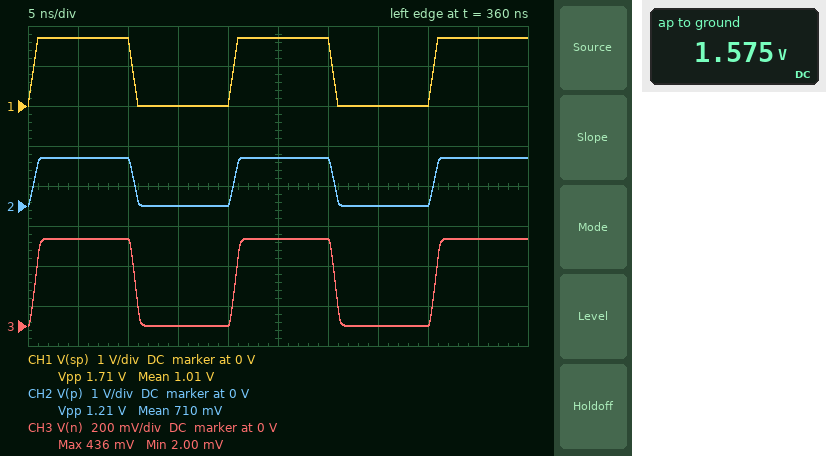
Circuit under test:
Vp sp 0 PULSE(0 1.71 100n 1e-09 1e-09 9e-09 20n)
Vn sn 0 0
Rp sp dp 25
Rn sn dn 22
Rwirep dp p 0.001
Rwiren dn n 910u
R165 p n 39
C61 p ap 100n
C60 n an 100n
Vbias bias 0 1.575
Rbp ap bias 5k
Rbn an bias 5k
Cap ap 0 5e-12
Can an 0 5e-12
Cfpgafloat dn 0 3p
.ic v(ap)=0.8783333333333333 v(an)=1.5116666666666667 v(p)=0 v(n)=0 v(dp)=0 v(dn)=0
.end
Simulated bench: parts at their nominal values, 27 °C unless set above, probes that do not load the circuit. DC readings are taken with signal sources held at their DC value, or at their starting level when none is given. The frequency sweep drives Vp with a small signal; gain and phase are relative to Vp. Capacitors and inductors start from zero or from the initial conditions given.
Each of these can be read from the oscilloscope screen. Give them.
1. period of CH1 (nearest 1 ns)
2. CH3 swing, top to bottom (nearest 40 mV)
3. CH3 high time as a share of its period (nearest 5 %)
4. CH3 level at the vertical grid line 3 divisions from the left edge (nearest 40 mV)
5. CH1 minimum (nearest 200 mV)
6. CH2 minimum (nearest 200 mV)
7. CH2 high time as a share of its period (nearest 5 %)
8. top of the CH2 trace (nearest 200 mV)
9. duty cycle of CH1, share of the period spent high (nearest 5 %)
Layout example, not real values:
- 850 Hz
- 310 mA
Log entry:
- 20 ns
- 440 mV
- 50 %
- 0 V
- 0 V
- 0 V
- 50 %
- 1.2 V
- 50 %
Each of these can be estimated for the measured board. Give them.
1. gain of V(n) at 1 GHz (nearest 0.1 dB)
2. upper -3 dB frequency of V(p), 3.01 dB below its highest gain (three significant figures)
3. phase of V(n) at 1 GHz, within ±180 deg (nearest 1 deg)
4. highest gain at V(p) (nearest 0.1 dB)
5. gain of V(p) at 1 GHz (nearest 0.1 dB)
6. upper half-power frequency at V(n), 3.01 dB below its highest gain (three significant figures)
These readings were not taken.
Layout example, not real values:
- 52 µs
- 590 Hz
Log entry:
- -15.4 dB
- 1.49 GHz
- -66 deg
- -3.0 dB
- -4.8 dB
- 901 MHz
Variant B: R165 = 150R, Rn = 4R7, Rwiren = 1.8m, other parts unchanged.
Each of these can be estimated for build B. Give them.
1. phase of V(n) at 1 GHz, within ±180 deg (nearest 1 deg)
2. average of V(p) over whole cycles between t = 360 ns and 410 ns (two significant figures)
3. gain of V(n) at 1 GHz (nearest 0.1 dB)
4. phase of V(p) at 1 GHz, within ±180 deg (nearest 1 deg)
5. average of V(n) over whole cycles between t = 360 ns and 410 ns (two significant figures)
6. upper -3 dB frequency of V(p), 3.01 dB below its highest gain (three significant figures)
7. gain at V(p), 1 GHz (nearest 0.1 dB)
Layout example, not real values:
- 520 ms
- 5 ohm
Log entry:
- -47 deg
- 740 mV
- -33.5 dB
- -34 deg
- 22 mV
- 1.48 GHz
- -3.0 dB
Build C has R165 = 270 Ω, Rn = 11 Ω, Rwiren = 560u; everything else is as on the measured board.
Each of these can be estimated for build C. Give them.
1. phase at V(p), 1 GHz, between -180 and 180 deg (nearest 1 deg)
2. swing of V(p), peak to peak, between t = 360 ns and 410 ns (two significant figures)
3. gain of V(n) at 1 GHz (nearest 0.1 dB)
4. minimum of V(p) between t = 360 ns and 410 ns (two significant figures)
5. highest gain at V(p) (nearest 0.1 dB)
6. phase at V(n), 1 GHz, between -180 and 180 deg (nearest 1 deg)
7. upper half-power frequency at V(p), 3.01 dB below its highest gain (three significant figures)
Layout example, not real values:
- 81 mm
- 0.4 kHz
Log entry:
- -36 deg
- 1.6 V
- -31.8 dB
- 3.2 mV
- -0.8 dB
- -64 deg
- 1.39 GHz
